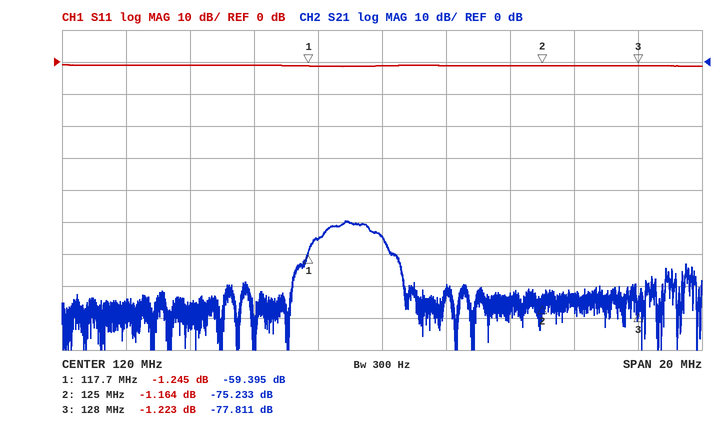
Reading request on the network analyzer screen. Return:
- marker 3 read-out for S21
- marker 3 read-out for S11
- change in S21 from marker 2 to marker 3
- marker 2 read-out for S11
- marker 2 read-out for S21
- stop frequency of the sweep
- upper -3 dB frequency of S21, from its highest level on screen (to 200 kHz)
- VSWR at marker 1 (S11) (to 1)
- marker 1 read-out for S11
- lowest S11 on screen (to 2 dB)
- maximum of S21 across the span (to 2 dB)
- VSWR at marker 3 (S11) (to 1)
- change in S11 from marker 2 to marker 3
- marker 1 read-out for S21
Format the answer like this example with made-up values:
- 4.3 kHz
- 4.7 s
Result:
- -77.811 dB
- -1.223 dB
- -2.578 dB
- -1.164 dB
- -75.233 dB
- 130 MHz
- 119.6 MHz
- 14
- -1.245 dB
- -2 dB
- -50 dB
- 14
- -0.059 dB
- -59.395 dB
